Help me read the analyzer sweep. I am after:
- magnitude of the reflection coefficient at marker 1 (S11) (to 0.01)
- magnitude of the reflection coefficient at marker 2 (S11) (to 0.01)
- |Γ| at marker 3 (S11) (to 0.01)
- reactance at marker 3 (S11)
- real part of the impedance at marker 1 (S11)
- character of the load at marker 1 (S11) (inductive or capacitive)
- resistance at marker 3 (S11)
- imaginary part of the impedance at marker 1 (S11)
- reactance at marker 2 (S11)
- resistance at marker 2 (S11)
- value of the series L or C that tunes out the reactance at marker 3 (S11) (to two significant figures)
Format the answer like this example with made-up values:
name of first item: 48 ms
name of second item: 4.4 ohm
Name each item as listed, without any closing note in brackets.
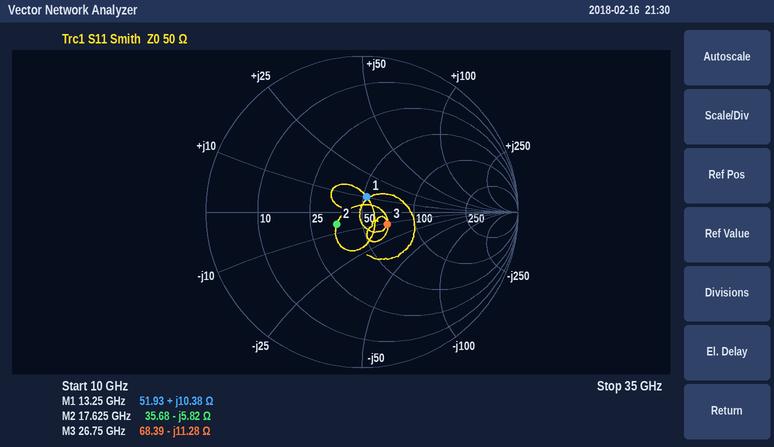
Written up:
magnitude of the reflection coefficient at marker 1 (S11): 0.10
magnitude of the reflection coefficient at marker 2 (S11): 0.18
|Γ| at marker 3 (S11): 0.18
reactance at marker 3: -11.28 Ω
real part of the impedance at marker 1: 51.93 Ω
character of the load at marker 1 (S11): inductive
resistance at marker 3: 68.39 Ω
imaginary part of the impedance at marker 1: +10.38 Ω
reactance at marker 2: -5.82 Ω
resistance at marker 2: 35.68 Ω
value of the series L or C that tunes out the reactance at marker 3 (S11): 67 pH
